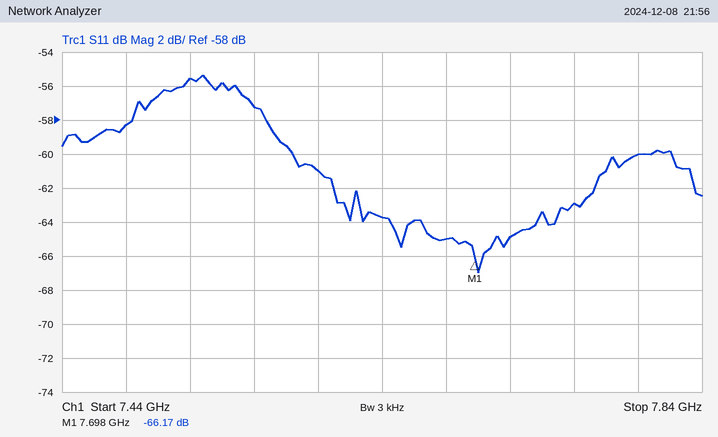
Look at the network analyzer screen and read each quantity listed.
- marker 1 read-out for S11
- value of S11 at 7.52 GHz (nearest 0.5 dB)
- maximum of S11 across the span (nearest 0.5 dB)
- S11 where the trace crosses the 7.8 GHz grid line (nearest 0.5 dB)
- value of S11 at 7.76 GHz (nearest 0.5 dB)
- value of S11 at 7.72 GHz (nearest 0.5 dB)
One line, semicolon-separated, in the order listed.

-66.17 dB; -55.5 dB; -55.5 dB; -60.0 dB; -63.0 dB; -65.0 dB
